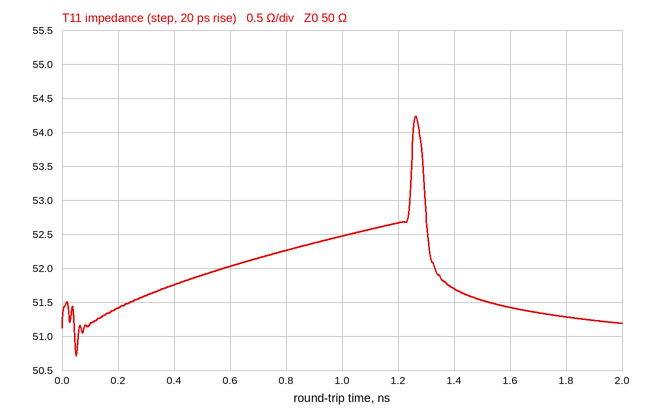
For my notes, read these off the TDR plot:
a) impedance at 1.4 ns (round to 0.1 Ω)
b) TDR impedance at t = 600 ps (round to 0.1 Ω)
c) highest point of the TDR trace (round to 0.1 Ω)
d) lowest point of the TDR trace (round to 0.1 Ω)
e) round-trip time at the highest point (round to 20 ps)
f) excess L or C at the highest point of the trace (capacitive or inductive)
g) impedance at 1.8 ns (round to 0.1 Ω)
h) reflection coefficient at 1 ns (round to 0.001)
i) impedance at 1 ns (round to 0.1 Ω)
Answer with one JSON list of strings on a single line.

["51.7 Ω", "52.0 Ω", "54.2 Ω", "50.7 Ω", "1.26 ns", "inductive", "51.3 Ω", "+0.024", "52.5 Ω"]
